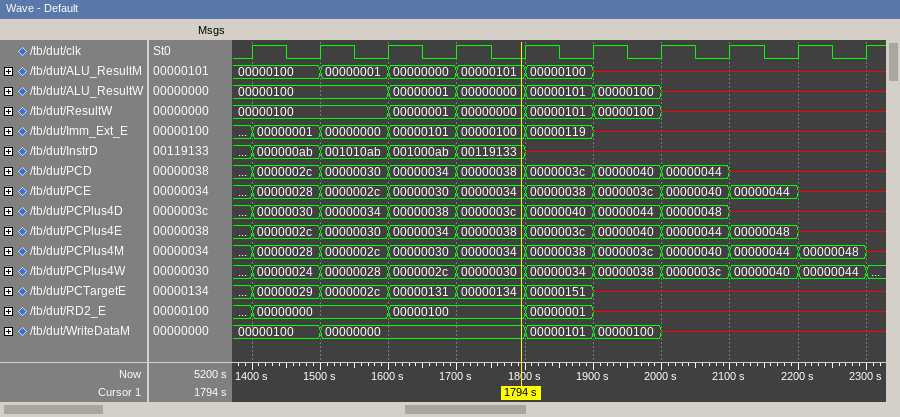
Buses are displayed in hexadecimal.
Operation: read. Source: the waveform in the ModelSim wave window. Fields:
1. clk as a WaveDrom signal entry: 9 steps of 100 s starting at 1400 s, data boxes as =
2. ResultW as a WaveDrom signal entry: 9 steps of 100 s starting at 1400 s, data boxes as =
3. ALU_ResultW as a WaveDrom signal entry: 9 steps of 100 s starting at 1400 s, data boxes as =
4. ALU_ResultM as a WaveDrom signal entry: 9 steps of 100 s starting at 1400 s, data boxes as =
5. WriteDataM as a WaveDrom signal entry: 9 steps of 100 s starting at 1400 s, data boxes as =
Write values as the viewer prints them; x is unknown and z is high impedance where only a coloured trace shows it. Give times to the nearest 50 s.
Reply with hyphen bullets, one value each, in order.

- {name: 'clk', wave: 'p........'}
- {name: 'ResultW', wave: '=.====x..', data: '00000100 00000001 00000000 00000101 00000100'}
- {name: 'ALU_ResultW', wave: '=.====x..', data: '00000100 00000001 00000000 00000101 00000100'}
- {name: 'ALU_ResultM', wave: '=====x...', data: '00000100 00000001 00000000 00000101 00000100'}
- {name: 'WriteDataM', wave: '==..==x..', data: '00000100 00000000 00000101 00000100'}
